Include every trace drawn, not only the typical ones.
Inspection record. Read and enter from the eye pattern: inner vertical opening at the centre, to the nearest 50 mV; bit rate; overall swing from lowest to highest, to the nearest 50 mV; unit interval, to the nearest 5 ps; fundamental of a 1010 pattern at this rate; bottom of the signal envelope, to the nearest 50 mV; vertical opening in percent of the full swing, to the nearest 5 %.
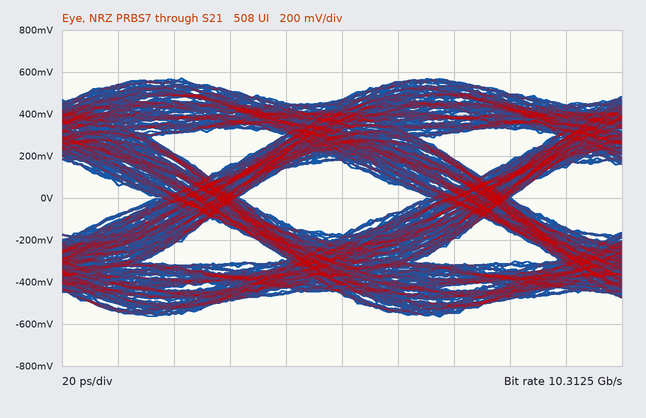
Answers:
350 mV
10.3125 Gb/s
1.15 V
95 ps
5.15625 GHz
-550 mV
30 %
